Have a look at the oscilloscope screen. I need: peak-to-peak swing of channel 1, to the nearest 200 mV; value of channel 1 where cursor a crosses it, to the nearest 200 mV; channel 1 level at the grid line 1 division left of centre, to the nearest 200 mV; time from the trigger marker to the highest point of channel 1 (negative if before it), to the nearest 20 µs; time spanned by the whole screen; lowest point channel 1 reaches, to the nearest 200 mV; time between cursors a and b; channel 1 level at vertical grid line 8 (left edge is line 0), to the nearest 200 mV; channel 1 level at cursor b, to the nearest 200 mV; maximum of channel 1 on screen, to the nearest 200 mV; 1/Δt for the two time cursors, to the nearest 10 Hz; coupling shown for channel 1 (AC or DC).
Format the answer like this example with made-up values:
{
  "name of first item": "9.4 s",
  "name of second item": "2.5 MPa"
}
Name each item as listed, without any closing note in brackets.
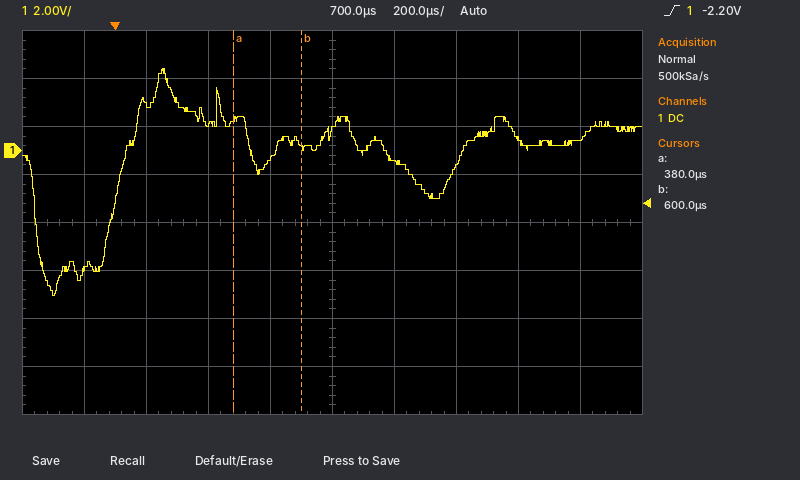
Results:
{
  "peak-to-peak swing of channel 1, to the nearest 200 mV": "9.4 V",
  "value of channel 1 where cursor a crosses it, to the nearest 200 mV": "1.2 V",
  "channel 1 level at the grid line 1 division left of centre, to the nearest 200 mV": "-400 mV",
  "time from the trigger marker to the highest point of channel 1 (negative if before it), to the nearest 20 µs": "+160 µs",
  "time spanned by the whole screen": "2 ms",
  "lowest point channel 1 reaches, to the nearest 200 mV": "-6.0 V",
  "time between cursors a and b": "220 µs",
  "channel 1 level at vertical grid line 8 (left edge is line 0), to the nearest 200 mV": "400 mV",
  "channel 1 level at cursor b, to the nearest 200 mV": "200 mV",
  "maximum of channel 1 on screen, to the nearest 200 mV": "3.4 V",
  "1/Δt for the two time cursors, to the nearest 10 Hz": "4.55 kHz",
  "coupling shown for channel 1": "DC"
}
